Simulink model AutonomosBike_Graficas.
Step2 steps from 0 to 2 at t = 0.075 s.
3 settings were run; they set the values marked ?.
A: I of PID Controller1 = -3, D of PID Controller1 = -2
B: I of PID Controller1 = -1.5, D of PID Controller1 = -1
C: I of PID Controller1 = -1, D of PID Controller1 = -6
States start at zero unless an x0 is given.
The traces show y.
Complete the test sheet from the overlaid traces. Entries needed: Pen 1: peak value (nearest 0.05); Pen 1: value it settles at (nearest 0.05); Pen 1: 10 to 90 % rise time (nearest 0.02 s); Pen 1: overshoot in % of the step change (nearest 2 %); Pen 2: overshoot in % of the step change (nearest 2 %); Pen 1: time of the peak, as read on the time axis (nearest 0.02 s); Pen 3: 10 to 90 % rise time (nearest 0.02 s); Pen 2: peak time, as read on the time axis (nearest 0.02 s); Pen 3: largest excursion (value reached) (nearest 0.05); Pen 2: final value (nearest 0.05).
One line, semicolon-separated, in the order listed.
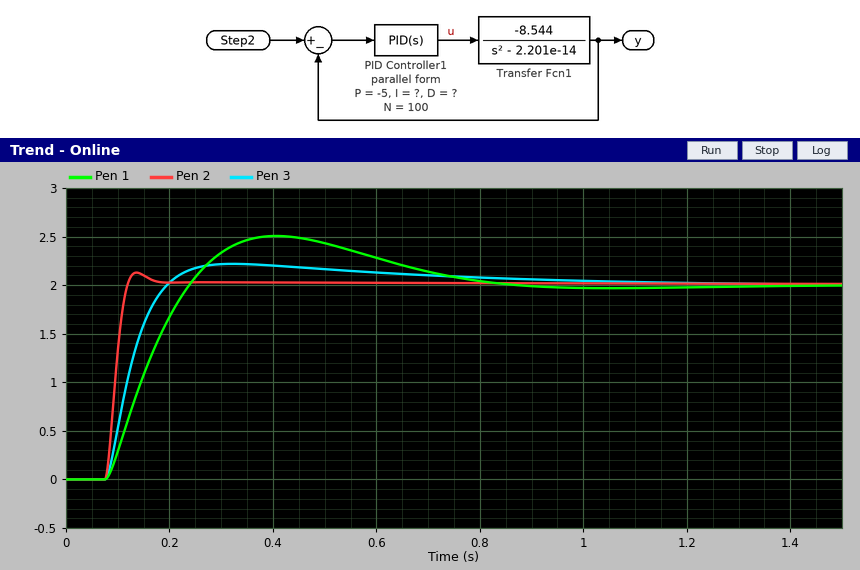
2.50; 2.00; 0.12 s; 26 %; 6 %; 0.40 s; 0.08 s; 0.14 s; 2.20; 2.00
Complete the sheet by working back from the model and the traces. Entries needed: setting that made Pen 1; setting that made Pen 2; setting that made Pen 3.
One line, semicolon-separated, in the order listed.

B; C; A
